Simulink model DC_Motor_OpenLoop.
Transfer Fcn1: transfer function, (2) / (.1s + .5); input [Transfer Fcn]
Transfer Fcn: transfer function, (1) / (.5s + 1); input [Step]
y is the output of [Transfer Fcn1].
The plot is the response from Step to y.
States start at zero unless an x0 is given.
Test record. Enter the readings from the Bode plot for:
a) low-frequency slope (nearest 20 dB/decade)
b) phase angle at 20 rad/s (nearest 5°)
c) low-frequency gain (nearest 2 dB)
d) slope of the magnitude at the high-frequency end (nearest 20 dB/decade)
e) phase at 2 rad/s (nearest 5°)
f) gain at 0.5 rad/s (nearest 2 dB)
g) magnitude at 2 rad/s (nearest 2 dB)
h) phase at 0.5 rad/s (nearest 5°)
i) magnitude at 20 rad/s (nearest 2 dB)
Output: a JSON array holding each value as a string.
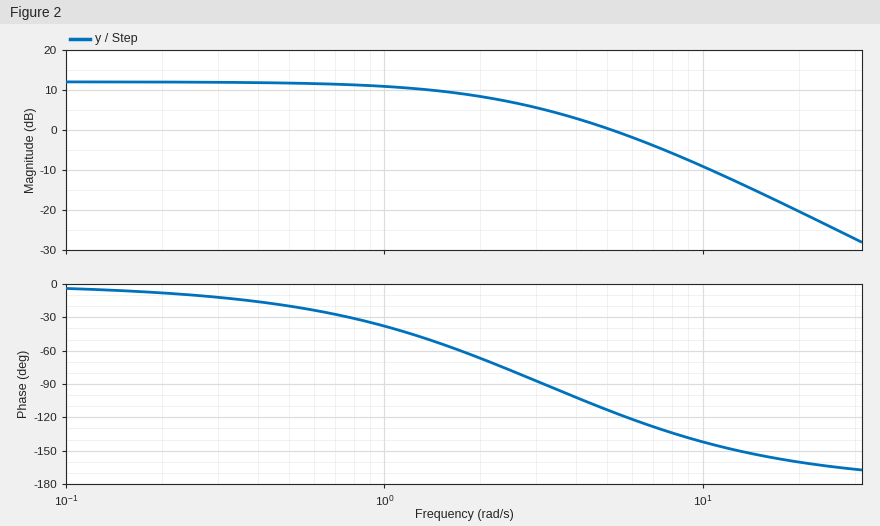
["0 dB/decade", "-160°", "12 dB", "-40 dB/decade", "-65°", "12 dB", "8 dB", "-20°", "-20 dB"]
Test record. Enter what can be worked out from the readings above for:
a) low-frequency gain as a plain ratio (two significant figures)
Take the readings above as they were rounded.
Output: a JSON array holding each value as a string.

["4.0"]
